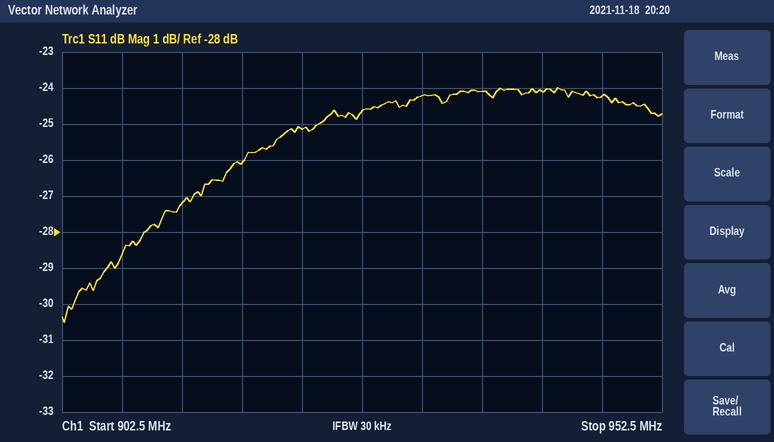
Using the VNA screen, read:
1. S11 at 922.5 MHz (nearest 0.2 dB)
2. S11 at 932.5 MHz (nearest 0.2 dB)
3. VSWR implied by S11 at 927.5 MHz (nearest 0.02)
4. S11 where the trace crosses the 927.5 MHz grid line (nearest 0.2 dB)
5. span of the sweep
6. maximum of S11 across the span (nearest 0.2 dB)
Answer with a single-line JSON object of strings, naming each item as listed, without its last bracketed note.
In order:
{"S11 at 922.5 MHz": "-25.2 dB", "S11 at 932.5 MHz": "-24.2 dB", "VSWR implied by S11 at 927.5 MHz": "1.12", "S11 where the trace crosses the 927.5 MHz grid line": "-24.6 dB", "span of the sweep": "50 MHz", "maximum of S11 across the span": "-24.0 dB"}
